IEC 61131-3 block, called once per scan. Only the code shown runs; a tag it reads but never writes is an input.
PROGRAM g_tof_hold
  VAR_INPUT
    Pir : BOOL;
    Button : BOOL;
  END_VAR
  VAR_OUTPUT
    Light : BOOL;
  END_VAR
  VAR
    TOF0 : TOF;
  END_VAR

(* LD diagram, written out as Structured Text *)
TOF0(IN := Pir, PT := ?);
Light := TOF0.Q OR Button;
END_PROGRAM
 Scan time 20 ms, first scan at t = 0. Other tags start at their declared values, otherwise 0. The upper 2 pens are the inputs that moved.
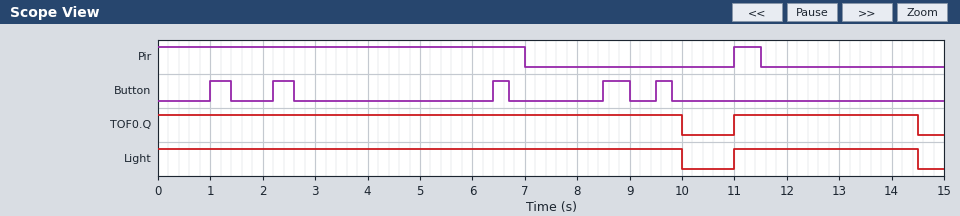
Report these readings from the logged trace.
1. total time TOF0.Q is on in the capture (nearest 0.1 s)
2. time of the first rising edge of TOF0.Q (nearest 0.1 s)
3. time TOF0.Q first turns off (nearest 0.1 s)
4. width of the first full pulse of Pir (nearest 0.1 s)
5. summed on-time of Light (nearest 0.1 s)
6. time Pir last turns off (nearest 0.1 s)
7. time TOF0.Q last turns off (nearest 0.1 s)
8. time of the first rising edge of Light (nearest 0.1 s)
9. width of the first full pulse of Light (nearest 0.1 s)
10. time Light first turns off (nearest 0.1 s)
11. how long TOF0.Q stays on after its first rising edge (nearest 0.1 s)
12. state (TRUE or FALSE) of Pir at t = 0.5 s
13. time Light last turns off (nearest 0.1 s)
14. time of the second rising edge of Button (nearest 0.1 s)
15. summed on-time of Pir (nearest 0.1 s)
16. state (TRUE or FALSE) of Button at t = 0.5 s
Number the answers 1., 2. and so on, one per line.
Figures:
1. 13.5 s
2. 11.0 s
3. 10.0 s
4. 0.5 s
5. 13.5 s
6. 11.5 s
7. 14.5 s
8. 11.0 s
9. 3.5 s
10. 10.0 s
11. 3.5 s
12. TRUE
13. 14.5 s
14. 2.2 s
15. 7.5 s
16. FALSE
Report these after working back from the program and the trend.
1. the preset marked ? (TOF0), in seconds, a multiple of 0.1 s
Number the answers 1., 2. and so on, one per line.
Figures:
1. 3.0 s
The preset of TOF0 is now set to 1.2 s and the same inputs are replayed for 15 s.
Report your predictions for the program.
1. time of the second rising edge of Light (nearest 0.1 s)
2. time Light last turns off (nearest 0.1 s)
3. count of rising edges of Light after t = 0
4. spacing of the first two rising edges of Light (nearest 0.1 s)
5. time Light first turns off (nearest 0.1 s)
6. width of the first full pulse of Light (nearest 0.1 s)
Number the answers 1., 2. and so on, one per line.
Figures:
1. 9.5 s
2. 12.7 s
3. 3
4. 1.0 s
5. 8.2 s
6. 0.5 s
